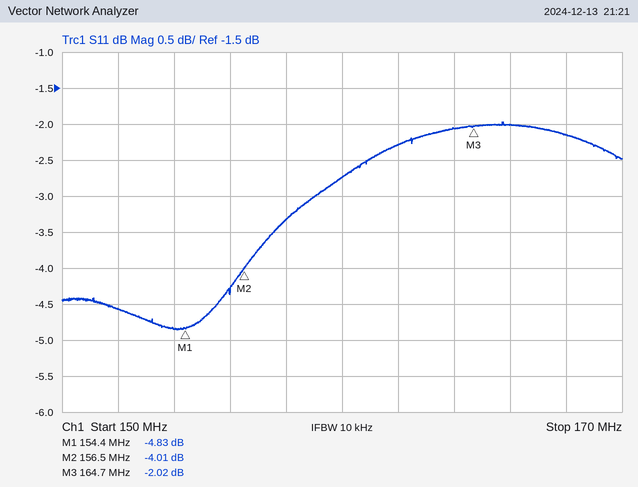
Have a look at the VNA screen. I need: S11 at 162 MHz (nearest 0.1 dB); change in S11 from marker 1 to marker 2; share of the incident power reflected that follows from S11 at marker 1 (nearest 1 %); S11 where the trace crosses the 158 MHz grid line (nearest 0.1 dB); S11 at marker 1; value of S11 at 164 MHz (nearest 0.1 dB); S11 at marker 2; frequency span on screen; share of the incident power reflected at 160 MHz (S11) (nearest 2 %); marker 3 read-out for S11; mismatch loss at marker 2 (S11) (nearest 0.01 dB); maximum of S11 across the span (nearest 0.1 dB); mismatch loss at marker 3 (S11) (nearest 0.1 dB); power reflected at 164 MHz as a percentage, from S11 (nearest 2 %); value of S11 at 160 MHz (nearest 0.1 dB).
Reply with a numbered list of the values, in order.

1. -2.3 dB
2. 0.82 dB
3. 33 %
4. -3.3 dB
5. -4.83 dB
6. -2.1 dB
7. -4.01 dB
8. 20 MHz
9. 54 %
10. -2.02 dB
11. 2.20 dB
12. -2.0 dB
13. 4.3 dB
14. 62 %
15. -2.7 dB
